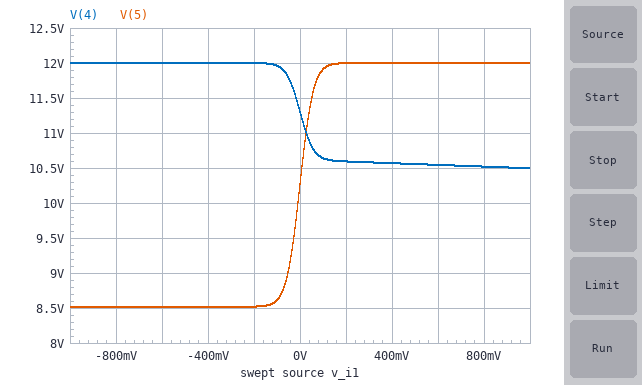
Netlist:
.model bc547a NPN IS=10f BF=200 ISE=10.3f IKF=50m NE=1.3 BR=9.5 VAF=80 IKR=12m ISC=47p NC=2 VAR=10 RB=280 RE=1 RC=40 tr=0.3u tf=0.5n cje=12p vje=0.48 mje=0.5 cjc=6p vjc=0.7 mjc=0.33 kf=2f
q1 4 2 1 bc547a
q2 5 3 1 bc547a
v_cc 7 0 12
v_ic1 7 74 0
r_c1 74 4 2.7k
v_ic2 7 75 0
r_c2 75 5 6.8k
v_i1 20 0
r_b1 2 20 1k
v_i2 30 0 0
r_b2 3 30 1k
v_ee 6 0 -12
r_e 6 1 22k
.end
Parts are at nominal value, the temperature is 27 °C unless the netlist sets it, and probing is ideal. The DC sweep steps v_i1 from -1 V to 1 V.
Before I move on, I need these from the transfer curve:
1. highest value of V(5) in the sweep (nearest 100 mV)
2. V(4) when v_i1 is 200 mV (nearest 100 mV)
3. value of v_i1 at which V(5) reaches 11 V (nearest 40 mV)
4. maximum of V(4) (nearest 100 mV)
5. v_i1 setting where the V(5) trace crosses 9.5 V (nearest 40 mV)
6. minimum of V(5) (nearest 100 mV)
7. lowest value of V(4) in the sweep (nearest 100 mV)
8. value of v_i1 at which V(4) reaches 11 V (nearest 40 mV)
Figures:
12.0 V
10.6 V
40 mV
12.0 V
-40 mV
8.5 V
10.5 V
40 mV
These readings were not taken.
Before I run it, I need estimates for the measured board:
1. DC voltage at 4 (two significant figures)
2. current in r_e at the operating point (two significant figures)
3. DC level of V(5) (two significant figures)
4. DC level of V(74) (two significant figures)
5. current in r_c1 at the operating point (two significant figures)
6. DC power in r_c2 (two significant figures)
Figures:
11 V
520 µA
10 V
12 V
260 µA
440 µW
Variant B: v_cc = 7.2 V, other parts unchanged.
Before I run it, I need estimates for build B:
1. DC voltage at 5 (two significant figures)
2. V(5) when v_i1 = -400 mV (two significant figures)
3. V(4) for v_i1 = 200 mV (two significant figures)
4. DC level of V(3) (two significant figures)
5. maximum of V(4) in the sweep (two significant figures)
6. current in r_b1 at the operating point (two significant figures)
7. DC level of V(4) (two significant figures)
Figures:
5.5 V
3.7 V
5.8 V
-2.3 mV
7.2 V
2.3 µA
6.5 V
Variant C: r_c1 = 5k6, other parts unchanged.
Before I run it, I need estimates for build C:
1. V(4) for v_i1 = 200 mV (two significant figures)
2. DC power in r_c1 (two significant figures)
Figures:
9.1 V
370 µW
